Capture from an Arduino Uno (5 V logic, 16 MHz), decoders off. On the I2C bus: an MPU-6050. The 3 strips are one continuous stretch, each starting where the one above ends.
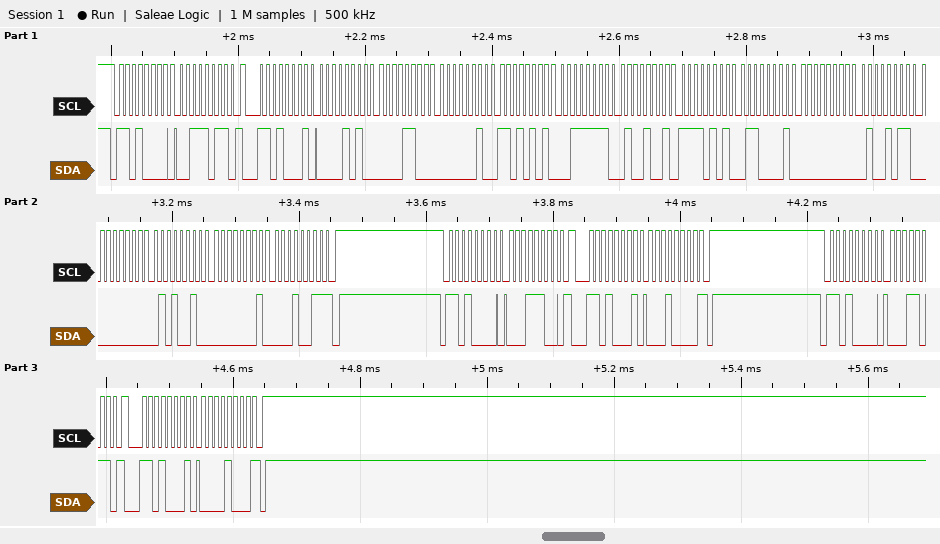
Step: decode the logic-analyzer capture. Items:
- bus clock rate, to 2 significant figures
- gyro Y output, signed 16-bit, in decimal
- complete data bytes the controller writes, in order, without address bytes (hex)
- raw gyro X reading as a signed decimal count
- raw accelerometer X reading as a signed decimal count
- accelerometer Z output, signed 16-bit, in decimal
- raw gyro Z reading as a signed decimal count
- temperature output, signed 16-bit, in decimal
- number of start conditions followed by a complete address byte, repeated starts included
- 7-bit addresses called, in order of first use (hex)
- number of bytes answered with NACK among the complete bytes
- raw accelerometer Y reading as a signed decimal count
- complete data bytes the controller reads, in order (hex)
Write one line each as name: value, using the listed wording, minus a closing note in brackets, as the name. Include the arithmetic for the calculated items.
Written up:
bus clock rate, to 2 significant figures: 100 kHz
gyro Y output, signed 16-bit, in decimal: 0x0052 = 82
complete data bytes the controller writes, in order, without address bytes: 3B 1C 1B
raw gyro X reading as a signed decimal count: 0x004B = 75
raw accelerometer X reading as a signed decimal count: 0x0A0C = 2572
accelerometer Z output, signed 16-bit, in decimal: 0x3F49 = 16201
raw gyro Z reading as a signed decimal count: 0x0113 = 275
temperature output, signed 16-bit, in decimal: 0xF561 = -2719
number of start conditions followed by a complete address byte, repeated starts included: 6
7-bit addresses called, in order of first use: 0x68
number of bytes answered with NACK among the complete bytes: 3
raw accelerometer Y reading as a signed decimal count: 0x02D5 = 725
complete data bytes the controller reads, in order: 0A 0C 02 D5 3F 49 F5 61 00 4B 00 52 01 13 10 08
